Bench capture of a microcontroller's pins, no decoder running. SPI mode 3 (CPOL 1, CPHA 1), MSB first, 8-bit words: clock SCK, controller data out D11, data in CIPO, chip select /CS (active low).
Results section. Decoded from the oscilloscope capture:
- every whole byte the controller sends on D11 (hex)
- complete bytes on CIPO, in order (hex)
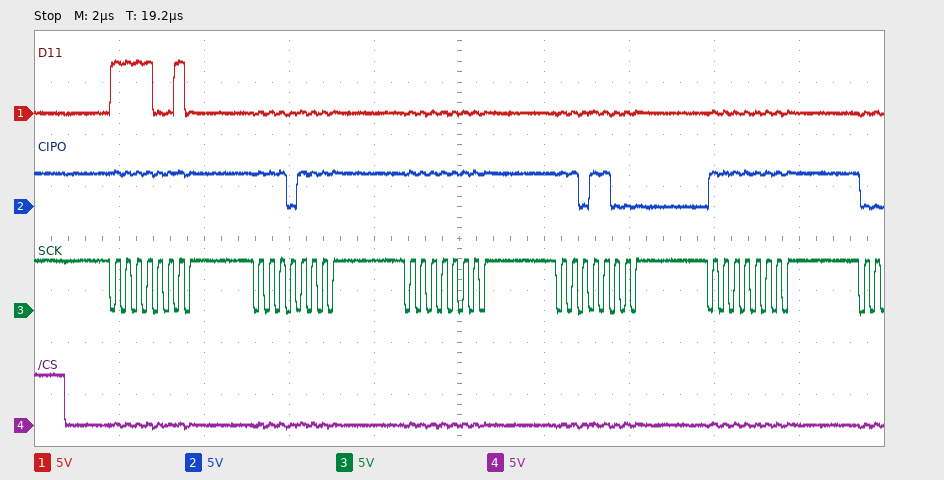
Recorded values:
F2 00 00 00 00
FF EF FF D8 FF
